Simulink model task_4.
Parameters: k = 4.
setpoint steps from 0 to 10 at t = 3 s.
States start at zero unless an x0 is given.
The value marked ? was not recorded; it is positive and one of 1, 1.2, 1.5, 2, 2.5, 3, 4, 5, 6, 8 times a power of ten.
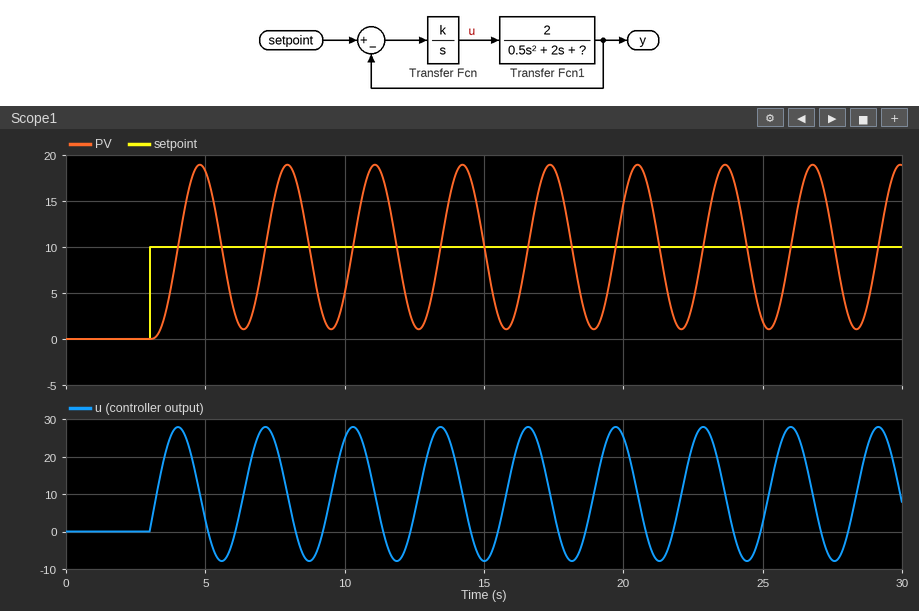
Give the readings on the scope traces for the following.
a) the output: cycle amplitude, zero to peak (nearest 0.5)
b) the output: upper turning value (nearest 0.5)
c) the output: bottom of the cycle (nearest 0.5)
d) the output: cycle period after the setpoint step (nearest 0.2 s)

9.0
19.0
1.0
3.2 s
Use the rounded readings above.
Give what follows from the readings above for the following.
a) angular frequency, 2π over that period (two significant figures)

2.0 rad/s
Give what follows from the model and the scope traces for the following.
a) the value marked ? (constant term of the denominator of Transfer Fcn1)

2
